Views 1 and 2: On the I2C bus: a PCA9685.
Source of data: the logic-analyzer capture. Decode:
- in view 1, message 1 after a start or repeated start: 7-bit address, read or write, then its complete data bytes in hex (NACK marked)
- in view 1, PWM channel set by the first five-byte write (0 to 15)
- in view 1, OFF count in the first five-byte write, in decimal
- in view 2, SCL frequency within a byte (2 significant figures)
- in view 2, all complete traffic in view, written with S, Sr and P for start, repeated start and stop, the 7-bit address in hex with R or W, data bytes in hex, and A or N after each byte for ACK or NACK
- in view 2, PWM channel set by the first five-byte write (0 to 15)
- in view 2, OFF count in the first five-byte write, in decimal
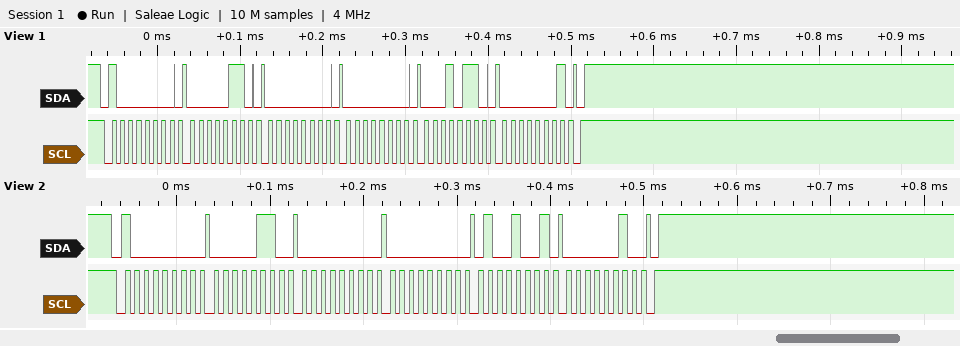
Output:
0x40 write: 06 00 00 16 01
0
278
100 kHz
S 40W A 06 A 00 A 00 A 49 A 02 A P
0
585
